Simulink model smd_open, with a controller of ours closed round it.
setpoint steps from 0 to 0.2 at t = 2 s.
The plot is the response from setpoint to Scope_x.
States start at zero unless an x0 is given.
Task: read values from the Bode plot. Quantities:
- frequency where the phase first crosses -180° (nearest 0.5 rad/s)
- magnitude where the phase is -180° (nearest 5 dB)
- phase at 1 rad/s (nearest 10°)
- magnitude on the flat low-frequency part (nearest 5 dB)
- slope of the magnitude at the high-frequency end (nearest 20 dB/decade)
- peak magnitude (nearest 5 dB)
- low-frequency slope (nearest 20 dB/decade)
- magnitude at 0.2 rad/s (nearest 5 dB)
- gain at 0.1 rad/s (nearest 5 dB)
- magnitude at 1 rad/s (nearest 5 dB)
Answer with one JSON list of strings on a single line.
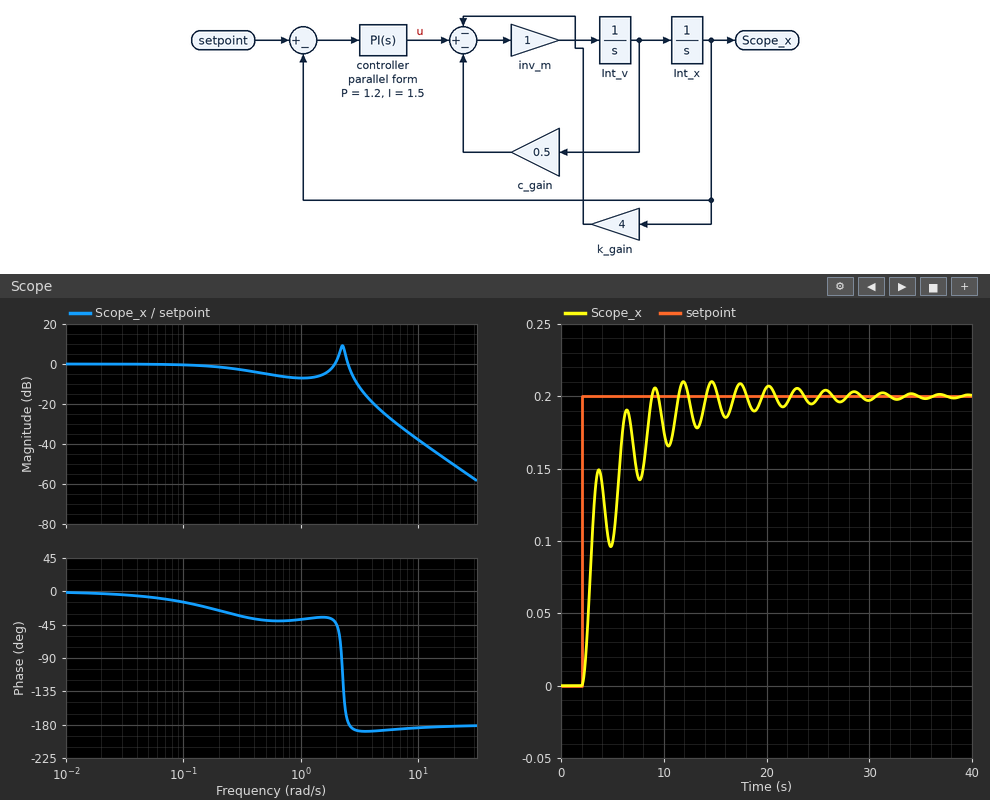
["2.5 rad/s", "0 dB", "-40°", "0 dB", "-40 dB/decade", "10 dB", "0 dB/decade", "0 dB", "0 dB", "-5 dB"]
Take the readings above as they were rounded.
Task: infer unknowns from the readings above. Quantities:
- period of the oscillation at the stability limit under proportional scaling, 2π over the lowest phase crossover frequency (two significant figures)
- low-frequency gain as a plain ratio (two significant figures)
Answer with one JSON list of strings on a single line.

["2.5 s", "1.0"]
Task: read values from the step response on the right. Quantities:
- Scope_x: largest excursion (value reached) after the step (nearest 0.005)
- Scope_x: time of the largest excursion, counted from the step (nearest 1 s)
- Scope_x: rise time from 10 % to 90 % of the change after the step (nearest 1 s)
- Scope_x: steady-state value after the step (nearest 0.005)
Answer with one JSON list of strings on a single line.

["0.210", "13 s", "4 s", "0.200"]
